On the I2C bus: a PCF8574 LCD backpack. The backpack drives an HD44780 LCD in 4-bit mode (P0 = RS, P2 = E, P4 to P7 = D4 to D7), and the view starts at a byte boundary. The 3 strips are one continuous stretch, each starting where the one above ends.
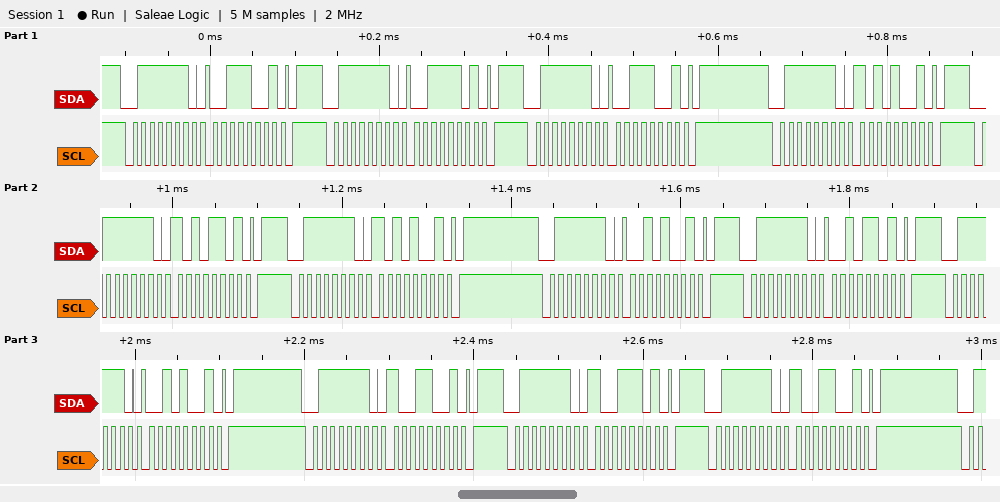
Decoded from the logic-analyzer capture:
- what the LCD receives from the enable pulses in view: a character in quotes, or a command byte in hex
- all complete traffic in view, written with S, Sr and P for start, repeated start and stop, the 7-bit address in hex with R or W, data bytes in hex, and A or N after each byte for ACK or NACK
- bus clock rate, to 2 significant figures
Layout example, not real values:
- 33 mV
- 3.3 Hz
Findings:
- ':' ')'
- S 3FW A 39 A P S 3FW A 3D A P S 3FW A 39 A P S 3FW A A9 A P S 3FW A AD A P S 3FW A A9 A P S 3FW A 29 A P S 3FW A 2D A P S 3FW A 29 A P S 3FW A 99 A P S 3FW A 9D A P S 3FW A 99 A P
- 100 kHz
